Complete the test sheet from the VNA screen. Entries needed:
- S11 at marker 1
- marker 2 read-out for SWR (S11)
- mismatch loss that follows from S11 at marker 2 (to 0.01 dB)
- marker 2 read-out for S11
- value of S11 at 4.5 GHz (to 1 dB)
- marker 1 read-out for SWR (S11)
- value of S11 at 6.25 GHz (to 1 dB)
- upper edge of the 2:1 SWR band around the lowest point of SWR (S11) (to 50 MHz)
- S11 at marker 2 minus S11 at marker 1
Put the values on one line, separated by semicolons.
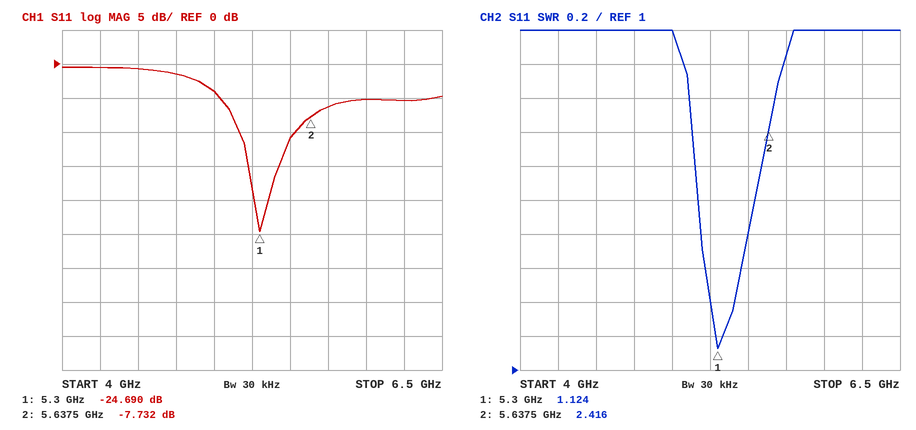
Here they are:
-24.690 dB; 2.416; 0.80 dB; -7.732 dB; -1 dB; 1.124; -5 dB; 5.55 GHz; 16.958 dB
